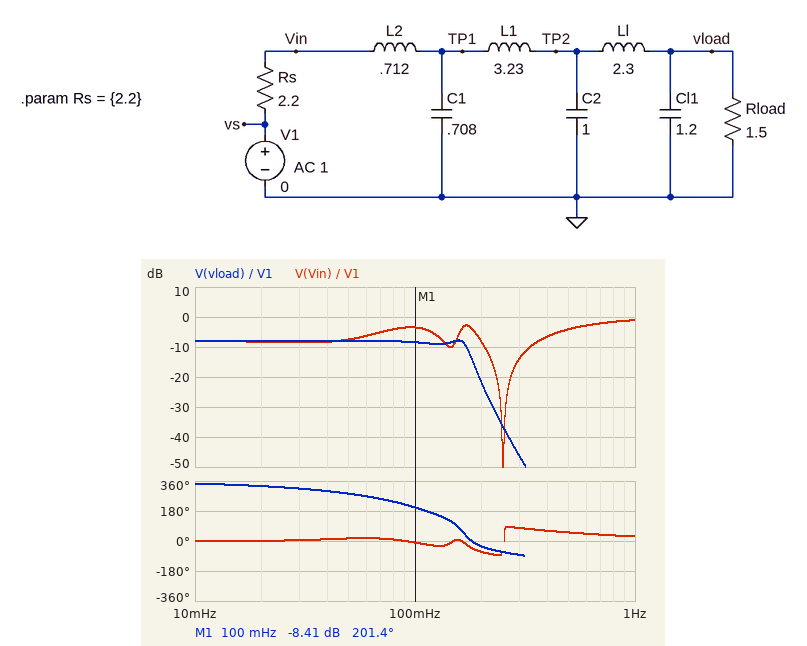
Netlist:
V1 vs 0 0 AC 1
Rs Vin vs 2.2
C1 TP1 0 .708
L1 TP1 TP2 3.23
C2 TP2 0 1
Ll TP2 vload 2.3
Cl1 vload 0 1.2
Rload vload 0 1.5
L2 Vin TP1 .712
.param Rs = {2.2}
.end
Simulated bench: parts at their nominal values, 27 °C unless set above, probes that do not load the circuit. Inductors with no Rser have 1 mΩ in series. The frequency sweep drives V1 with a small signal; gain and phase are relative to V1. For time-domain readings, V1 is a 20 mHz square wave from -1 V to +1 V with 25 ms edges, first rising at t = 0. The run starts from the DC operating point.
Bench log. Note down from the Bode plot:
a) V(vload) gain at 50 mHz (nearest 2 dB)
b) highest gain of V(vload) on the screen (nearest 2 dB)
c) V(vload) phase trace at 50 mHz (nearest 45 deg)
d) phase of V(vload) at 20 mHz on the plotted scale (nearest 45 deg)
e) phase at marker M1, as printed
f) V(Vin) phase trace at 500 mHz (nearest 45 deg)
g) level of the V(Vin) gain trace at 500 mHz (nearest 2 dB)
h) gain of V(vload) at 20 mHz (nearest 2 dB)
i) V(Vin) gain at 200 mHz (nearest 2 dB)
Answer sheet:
-8 dB
-8 dB
270 deg
315 deg
201.4 deg
45 deg
-4 dB
-8 dB
-8 dB
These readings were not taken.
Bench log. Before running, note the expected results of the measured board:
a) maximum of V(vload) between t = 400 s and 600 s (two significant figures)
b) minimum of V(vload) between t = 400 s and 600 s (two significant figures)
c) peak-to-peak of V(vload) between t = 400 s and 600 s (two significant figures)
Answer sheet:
510 mV
-510 mV
1.0 V
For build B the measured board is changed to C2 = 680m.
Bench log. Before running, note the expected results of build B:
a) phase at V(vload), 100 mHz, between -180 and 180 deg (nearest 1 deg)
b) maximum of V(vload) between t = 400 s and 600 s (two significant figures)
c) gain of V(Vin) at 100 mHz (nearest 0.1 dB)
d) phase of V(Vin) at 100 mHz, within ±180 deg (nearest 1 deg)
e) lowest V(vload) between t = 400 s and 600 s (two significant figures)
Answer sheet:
-151 deg
470 mV
-2.8 dB
-11 deg
-470 mV
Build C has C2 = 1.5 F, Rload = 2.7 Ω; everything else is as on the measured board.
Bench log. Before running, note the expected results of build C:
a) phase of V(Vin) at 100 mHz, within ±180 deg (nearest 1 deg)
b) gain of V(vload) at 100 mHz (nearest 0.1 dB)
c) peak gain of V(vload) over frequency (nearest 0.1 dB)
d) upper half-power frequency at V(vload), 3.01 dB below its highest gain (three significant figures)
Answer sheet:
0 deg
-6.1 dB
-5.2 dB
152 mHz
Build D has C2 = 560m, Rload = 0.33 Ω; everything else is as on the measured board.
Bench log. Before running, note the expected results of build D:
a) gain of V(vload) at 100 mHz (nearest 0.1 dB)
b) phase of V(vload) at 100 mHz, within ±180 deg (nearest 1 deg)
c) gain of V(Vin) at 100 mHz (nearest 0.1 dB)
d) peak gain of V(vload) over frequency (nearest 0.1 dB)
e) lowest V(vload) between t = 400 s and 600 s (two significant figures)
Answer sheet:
-18.8 dB
-130 deg
-2.1 dB
-14.7 dB
-160 mV
